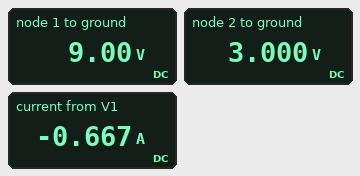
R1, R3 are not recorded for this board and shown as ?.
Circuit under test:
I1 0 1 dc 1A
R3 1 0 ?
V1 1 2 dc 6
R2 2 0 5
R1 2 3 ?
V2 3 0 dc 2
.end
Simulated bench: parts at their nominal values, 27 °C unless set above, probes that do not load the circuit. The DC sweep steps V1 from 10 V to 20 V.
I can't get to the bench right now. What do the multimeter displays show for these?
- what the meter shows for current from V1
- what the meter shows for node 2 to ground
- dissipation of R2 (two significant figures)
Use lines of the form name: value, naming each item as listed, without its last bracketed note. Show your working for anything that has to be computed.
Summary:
what the meter shows for current from V1: -0.667 A
what the meter shows for node 2 to ground: 3.000 V
dissipation of R2: (3 V)^2 / 5 Ω = 1.8 W
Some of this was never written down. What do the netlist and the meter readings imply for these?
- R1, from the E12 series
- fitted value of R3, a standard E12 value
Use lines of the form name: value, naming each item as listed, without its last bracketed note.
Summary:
R1, from the E12 series: 15 Ω
fitted value of R3, a standard E12 value: 27 Ω
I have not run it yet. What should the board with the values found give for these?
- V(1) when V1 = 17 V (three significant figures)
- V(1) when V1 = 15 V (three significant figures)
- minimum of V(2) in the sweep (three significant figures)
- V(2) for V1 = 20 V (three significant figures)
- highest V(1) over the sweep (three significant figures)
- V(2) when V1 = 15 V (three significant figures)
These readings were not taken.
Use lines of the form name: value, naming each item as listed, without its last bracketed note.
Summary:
V(1) when V1 = 17 V: 18.7 V
V(1) when V1 = 15 V: 16.9 V
minimum of V(2) in the sweep: 1.29 V
V(2) for V1 = 20 V: 1.29 V
highest V(1) over the sweep: 21.3 V
V(2) when V1 = 15 V: 1.90 V
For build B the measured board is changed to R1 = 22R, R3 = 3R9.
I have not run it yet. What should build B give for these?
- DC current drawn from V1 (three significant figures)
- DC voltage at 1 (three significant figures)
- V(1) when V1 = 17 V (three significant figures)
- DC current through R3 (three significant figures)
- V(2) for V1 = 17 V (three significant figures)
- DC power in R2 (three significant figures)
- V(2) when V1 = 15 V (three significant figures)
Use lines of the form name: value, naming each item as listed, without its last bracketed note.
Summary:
DC current drawn from V1: 310 mA
DC voltage at 1: 5.11 V
V(1) when V1 = 17 V: 10.5 V
DC current through R3: 1.31 A
V(2) for V1 = 17 V: -6.51 V
DC power in R2: 159 mW
V(2) when V1 = 15 V: -5.49 V
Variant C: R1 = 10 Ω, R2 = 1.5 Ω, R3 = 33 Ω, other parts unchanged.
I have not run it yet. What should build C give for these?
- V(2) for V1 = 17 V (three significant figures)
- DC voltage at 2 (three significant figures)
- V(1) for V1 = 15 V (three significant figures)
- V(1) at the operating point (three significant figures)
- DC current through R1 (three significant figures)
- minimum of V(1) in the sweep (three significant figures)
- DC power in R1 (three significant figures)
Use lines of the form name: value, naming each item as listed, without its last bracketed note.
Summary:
V(2) for V1 = 17 V: 859 mV
DC voltage at 2: 1.28 V
V(1) for V1 = 15 V: 15.9 V
V(1) at the operating point: 7.28 V
DC current through R1: 72.2 mA
minimum of V(1) in the sweep: 11.1 V
DC power in R1: 52.2 mW
